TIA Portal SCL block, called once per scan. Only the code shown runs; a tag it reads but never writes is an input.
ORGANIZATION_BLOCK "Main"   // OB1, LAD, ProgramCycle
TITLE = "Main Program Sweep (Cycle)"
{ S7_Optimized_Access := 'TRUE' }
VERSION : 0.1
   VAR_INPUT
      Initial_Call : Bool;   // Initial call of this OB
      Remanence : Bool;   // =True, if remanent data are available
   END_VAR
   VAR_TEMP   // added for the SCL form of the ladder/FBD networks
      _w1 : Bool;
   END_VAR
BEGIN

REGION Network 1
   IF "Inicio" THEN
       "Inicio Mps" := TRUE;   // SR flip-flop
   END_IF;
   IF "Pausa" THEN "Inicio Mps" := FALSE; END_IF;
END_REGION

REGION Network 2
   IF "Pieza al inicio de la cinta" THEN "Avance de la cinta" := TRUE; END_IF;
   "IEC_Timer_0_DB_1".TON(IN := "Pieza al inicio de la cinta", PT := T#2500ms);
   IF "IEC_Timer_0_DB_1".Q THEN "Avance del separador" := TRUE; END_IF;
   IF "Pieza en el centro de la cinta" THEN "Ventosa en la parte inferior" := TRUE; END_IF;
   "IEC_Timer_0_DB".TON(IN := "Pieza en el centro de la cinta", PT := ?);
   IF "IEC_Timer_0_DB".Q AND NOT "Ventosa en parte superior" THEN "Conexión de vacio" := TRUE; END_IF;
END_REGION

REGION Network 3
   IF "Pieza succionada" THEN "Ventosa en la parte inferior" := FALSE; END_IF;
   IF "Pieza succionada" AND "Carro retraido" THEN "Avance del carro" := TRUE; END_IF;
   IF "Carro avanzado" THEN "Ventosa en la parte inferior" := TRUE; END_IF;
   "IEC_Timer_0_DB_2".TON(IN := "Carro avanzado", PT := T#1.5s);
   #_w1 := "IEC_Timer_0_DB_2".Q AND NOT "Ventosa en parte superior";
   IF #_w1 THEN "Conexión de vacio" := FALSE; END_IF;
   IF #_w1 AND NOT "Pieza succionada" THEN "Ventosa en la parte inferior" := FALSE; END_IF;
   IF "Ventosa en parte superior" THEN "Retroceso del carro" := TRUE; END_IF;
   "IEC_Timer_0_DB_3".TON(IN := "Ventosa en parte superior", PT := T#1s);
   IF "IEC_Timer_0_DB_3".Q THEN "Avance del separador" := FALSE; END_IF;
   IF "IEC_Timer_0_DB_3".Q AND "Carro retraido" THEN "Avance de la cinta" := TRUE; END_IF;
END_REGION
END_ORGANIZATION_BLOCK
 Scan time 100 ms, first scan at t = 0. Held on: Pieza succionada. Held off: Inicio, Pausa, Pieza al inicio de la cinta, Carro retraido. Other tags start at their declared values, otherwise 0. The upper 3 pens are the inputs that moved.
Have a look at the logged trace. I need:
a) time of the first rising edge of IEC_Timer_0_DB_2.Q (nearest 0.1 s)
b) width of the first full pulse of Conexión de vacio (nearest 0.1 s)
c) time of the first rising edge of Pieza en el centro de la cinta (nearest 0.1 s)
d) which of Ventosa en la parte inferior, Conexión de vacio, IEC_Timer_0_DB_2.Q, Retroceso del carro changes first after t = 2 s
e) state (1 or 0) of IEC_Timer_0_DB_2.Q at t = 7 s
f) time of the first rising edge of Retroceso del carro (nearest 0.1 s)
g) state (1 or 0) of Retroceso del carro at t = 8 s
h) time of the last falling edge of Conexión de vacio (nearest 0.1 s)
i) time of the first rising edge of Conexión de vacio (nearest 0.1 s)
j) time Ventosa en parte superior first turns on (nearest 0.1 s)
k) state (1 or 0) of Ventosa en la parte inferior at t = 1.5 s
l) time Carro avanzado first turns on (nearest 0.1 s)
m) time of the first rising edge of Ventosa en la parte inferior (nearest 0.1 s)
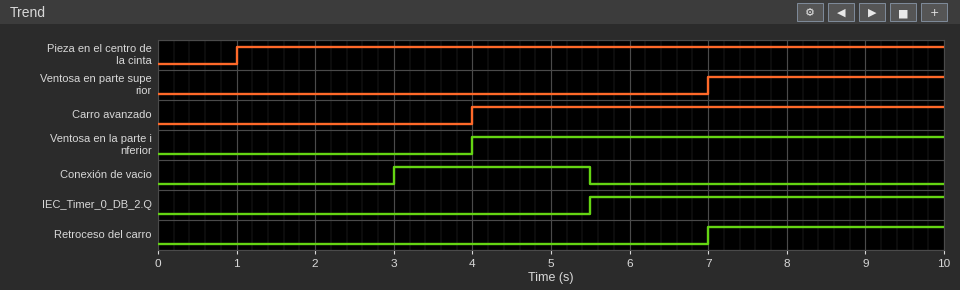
5.5 s
2.5 s
1.0 s
Conexión de vacio
1
7.0 s
1
5.5 s
3.0 s
7.0 s
0
4.0 s
4.0 s
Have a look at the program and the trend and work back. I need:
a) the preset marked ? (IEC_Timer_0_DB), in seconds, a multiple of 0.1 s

2.0 s
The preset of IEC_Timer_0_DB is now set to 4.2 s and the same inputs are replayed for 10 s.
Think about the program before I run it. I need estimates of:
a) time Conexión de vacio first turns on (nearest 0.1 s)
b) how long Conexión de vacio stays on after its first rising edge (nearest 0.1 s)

5.2 s
0.3 s
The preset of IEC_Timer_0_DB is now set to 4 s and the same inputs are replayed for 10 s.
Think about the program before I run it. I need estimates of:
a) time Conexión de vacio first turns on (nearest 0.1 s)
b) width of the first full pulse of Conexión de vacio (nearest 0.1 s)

5.0 s
0.5 s
